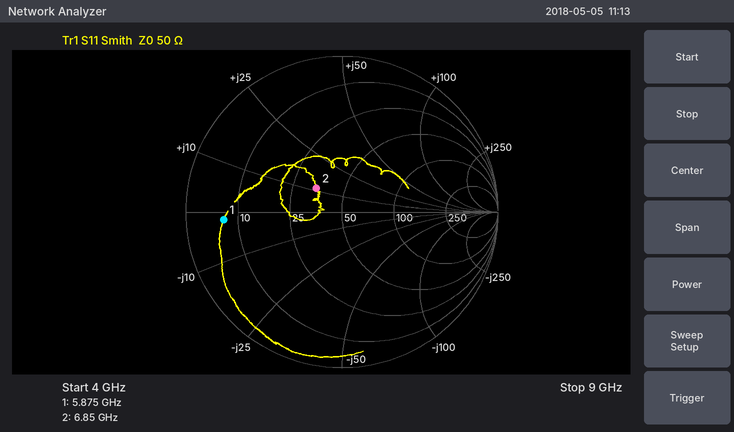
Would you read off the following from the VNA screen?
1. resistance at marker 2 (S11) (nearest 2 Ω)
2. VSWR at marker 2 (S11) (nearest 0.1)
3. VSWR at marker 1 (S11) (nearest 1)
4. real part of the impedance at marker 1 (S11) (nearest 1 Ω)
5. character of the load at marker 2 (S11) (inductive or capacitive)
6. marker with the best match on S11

34 Ω
1.6
7
7 Ω
inductive
marker 2
